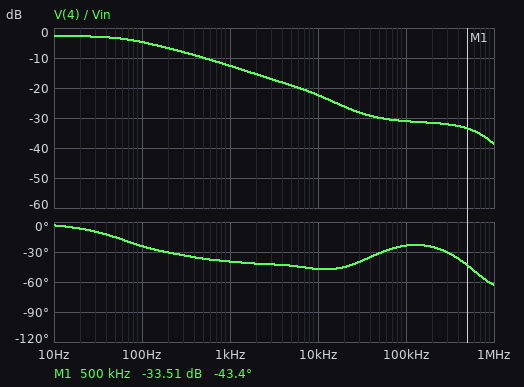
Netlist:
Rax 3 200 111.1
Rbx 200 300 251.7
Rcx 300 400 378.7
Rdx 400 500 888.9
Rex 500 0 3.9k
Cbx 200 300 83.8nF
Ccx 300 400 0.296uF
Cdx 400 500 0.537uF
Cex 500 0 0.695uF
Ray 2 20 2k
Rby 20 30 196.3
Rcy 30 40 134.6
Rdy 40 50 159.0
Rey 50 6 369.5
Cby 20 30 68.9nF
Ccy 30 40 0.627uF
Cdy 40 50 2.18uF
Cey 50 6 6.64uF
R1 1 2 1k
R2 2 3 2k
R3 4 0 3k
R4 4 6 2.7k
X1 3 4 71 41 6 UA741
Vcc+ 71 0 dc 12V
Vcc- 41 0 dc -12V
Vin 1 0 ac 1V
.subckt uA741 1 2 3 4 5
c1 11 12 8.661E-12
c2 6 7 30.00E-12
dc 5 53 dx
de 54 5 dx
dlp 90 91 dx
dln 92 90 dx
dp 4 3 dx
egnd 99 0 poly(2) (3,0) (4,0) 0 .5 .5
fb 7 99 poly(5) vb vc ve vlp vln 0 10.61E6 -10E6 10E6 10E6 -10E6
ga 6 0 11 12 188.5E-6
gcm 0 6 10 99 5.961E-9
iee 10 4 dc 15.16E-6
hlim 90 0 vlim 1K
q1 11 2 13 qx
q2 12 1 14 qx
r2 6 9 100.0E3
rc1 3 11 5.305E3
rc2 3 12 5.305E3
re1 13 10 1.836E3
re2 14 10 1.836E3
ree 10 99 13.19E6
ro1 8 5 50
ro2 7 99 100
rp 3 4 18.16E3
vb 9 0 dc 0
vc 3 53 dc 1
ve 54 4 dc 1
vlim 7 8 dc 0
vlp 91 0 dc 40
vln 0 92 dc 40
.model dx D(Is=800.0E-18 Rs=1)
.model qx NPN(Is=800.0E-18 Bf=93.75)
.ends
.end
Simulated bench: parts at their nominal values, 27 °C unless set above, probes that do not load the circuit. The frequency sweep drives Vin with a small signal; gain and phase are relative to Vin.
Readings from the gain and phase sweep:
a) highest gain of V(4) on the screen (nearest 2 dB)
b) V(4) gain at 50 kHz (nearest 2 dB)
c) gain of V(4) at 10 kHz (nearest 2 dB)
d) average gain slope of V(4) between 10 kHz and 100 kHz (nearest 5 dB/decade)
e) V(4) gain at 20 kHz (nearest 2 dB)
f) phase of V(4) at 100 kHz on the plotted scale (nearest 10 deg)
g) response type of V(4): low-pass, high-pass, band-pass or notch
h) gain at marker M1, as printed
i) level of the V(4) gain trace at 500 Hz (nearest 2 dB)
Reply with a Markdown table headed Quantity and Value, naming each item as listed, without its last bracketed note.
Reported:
| Quantity | Value |
|---|---|
| highest gain of V(4) on the screen | -2 dB |
| V(4) gain at 50 kHz | -30 dB |
| gain of V(4) at 10 kHz | -22 dB |
| average gain slope of V(4) between 10 kHz and 100 kHz | -10 dB/decade |
| V(4) gain at 20 kHz | -26 dB |
| phase of V(4) at 100 kHz on the plotted scale | -20 deg |
| response type of V(4): low-pass, high-pass, band-pass or notch | low-pass |
| gain at marker M1, as printed | -33.51 dB |
| level of the V(4) gain trace at 500 Hz | -10 dB |
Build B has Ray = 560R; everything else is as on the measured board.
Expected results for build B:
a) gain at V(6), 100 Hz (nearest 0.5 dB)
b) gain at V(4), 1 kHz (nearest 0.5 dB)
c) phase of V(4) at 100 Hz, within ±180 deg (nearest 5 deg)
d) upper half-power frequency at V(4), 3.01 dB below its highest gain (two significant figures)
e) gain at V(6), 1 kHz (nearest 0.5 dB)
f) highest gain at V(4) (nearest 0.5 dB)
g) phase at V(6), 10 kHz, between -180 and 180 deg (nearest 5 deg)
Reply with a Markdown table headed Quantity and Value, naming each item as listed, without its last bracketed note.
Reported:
| Quantity | Value |
|---|---|
| gain at V(6), 100 Hz | 1.5 dB |
| gain at V(4), 1 kHz | -14.0 dB |
| phase of V(4) at 100 Hz, within ±180 deg | -30 deg |
| upper half-power frequency at V(4), 3.01 dB below its highest gain | 110 Hz |
| gain at V(6), 1 kHz | -8.5 dB |
| highest gain at V(4) | -1.5 dB |
| phase at V(6), 10 kHz, between -180 and 180 deg | -55 deg |
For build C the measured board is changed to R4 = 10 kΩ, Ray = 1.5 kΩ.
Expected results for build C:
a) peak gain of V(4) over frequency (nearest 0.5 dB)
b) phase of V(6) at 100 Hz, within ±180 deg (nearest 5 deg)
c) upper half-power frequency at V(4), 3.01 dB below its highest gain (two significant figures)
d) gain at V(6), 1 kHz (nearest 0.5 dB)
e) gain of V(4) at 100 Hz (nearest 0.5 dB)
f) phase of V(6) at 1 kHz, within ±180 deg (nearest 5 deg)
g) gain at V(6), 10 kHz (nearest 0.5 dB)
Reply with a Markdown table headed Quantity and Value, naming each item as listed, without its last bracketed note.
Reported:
| Quantity | Value |
|---|---|
| peak gain of V(4) over frequency | 11.0 dB |
| phase of V(6) at 100 Hz, within ±180 deg | -60 deg |
| upper half-power frequency at V(4), 3.01 dB below its highest gain | 47 Hz |
| gain at V(6), 1 kHz | 2.0 dB |
| gain of V(4) at 100 Hz | 3.0 dB |
| phase of V(6) at 1 kHz, within ±180 deg | -55 deg |
| gain at V(6), 10 kHz | -9.5 dB |
